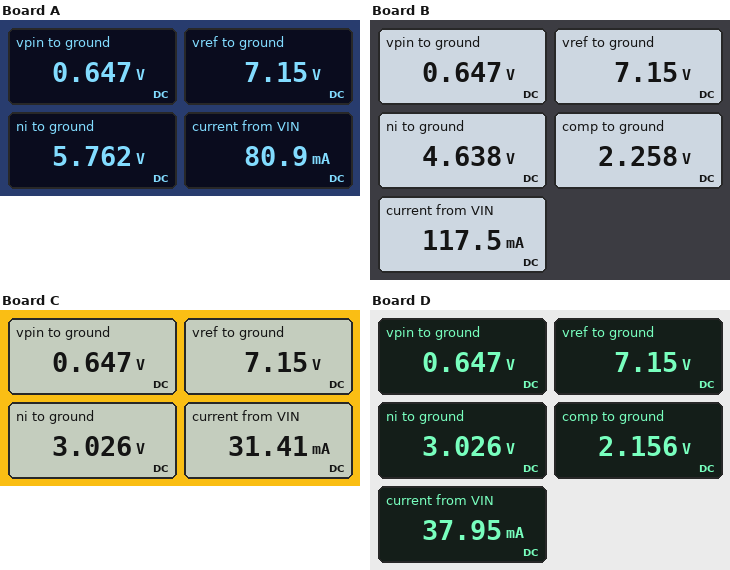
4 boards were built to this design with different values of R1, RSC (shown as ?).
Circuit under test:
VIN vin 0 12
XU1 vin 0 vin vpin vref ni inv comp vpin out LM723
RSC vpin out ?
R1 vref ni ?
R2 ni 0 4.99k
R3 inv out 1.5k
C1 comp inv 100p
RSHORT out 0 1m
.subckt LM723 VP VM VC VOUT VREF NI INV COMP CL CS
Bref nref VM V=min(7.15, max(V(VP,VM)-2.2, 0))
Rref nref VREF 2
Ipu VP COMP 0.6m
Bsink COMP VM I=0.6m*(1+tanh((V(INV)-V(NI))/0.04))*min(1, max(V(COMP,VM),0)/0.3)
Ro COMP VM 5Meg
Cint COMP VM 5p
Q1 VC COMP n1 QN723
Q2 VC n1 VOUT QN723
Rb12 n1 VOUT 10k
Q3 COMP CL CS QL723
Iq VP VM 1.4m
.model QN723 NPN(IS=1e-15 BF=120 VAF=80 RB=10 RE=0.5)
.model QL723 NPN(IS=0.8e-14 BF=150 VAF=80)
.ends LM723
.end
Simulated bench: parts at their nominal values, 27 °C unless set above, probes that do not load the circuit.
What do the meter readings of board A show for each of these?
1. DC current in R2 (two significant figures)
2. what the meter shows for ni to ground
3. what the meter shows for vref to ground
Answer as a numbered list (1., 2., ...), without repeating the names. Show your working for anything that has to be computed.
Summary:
1. (5.762 V) / 4.99 kΩ = 1.2 mA
2. 5.762 V
3. 7.15 V
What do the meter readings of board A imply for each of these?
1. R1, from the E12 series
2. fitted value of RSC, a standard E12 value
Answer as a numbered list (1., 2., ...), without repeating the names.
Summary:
1. 1.2 kΩ
2. 8.2 Ω
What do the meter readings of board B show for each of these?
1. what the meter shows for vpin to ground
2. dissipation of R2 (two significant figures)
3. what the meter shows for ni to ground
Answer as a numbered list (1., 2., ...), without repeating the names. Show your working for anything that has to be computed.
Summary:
1. 0.647 V
2. (4.638 V)^2 / 4.99 kΩ = 4.3 mW
3. 4.638 V
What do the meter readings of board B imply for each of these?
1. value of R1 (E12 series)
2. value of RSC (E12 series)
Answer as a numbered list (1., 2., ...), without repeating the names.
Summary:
1. 2.7 kΩ
2. 5.6 Ω
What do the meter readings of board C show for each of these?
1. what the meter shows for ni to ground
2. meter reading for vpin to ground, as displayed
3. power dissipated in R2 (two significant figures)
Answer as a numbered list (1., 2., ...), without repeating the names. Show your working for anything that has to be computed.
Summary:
1. 3.026 V
2. 0.647 V
3. (3.026 V)^2 / 4.99 kΩ = 1.8 mW
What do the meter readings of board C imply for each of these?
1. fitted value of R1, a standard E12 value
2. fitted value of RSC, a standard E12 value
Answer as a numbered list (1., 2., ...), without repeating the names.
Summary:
1. 6.8 kΩ
2. 22 Ω
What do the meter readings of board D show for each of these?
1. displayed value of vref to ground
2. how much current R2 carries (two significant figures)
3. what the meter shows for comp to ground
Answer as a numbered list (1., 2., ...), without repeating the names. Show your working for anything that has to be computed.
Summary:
1. 7.15 V
2. (3.026 V) / 4.99 kΩ = 610 µA
3. 2.156 V
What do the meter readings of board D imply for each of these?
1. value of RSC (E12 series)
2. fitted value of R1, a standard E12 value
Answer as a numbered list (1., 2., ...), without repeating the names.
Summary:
1. 18 Ω
2. 6.8 kΩ
